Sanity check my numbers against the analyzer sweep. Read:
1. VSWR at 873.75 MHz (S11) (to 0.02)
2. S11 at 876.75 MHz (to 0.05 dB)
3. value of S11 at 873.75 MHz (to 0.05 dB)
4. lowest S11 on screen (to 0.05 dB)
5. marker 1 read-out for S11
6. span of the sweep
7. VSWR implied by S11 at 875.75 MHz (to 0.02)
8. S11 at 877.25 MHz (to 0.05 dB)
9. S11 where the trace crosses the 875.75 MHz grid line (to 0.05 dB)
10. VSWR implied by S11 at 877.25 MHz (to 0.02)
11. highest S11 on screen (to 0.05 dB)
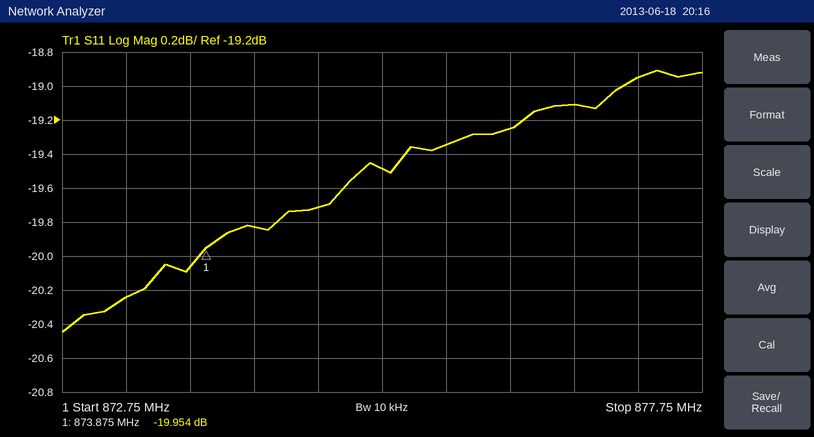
1.22
-19.10 dB
-20.05 dB
-20.45 dB
-19.954 dB
5 MHz
1.24
-18.95 dB
-19.35 dB
1.26
-18.90 dB
